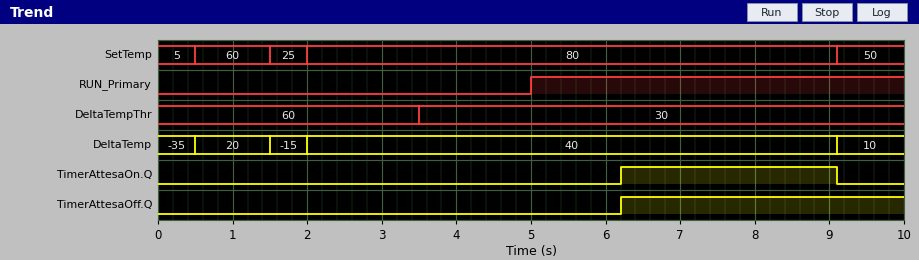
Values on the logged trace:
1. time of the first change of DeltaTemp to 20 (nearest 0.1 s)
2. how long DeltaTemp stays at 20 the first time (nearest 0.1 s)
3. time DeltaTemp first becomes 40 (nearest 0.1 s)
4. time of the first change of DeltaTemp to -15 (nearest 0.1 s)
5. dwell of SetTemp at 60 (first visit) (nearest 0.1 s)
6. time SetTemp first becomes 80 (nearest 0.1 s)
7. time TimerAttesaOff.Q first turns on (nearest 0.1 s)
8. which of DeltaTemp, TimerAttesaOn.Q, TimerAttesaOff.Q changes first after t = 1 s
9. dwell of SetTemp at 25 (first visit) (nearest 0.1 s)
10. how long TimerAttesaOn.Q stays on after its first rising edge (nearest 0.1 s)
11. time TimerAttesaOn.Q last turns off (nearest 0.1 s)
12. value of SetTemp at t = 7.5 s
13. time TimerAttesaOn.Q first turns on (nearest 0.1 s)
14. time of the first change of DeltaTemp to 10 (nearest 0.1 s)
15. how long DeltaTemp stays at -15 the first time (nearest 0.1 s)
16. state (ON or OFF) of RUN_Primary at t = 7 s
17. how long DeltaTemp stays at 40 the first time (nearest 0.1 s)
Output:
0.5 s
1.0 s
2.0 s
1.5 s
1.0 s
2.0 s
6.2 s
DeltaTemp
0.5 s
2.9 s
9.1 s
80
6.2 s
9.1 s
0.5 s
ON
7.1 s
